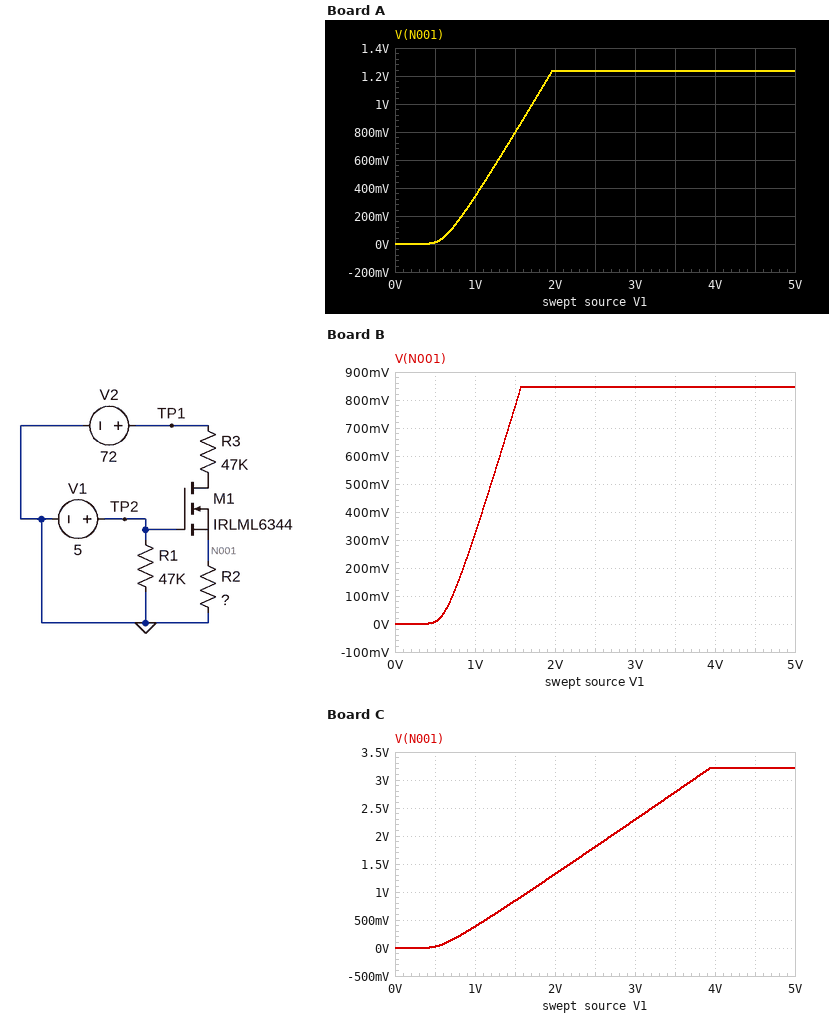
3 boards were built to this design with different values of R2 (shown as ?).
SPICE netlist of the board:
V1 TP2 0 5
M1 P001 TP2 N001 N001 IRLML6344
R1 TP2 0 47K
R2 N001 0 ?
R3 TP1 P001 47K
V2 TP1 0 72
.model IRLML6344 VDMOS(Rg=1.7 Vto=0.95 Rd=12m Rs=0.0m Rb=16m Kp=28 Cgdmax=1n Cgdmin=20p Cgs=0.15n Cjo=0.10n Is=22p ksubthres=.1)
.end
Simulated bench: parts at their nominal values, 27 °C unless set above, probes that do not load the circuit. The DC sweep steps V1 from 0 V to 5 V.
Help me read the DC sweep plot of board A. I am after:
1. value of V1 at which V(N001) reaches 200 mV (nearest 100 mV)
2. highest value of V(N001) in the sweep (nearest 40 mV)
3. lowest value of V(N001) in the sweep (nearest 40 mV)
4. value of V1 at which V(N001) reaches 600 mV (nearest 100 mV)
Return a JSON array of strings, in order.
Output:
["800 mV", "1.24 V", "0 V", "1.3 V"]
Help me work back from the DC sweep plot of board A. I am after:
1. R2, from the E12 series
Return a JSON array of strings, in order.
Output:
["820 Ω"]
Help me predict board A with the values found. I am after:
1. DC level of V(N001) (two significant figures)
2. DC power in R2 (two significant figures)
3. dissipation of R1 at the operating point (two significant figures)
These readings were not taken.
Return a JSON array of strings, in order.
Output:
["1.2 V", "1.9 mW", "530 µW"]
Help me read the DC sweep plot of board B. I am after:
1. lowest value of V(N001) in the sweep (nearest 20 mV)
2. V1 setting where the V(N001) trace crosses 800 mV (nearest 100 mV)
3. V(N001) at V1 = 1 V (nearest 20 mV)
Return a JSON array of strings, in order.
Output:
["0 V", "1.5 V", "320 mV"]
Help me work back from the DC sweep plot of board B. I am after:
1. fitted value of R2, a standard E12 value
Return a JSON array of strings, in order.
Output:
["560 Ω"]
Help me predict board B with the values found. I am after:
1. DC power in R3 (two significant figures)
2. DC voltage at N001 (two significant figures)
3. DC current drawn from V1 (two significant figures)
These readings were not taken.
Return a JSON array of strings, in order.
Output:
["110 mW", "850 mV", "110 µA"]
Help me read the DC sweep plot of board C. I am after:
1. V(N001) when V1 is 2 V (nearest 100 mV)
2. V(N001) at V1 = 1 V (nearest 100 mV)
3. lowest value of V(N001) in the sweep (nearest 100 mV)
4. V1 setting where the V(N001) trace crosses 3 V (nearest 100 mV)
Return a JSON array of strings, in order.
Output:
["1.3 V", "400 mV", "0 V", "3.7 V"]
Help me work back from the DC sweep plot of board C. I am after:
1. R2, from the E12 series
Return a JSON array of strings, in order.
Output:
["2.2 kΩ"]
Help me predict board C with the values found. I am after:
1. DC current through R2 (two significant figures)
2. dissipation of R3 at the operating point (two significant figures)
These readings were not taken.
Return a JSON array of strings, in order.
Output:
["1.5 mA", "100 mW"]
